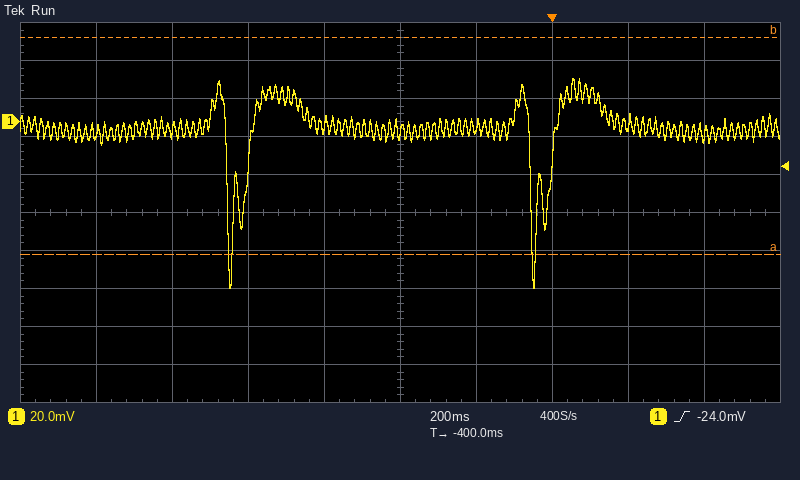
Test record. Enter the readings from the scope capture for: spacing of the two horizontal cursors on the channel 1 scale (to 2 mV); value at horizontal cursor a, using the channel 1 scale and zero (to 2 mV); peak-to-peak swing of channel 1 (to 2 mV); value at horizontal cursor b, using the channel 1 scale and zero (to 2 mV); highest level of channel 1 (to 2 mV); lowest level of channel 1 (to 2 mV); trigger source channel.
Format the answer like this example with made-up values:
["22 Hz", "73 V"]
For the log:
["114 mV", "-70 mV", "110 mV", "44 mV", "22 mV", "-88 mV", "channel 1"]
